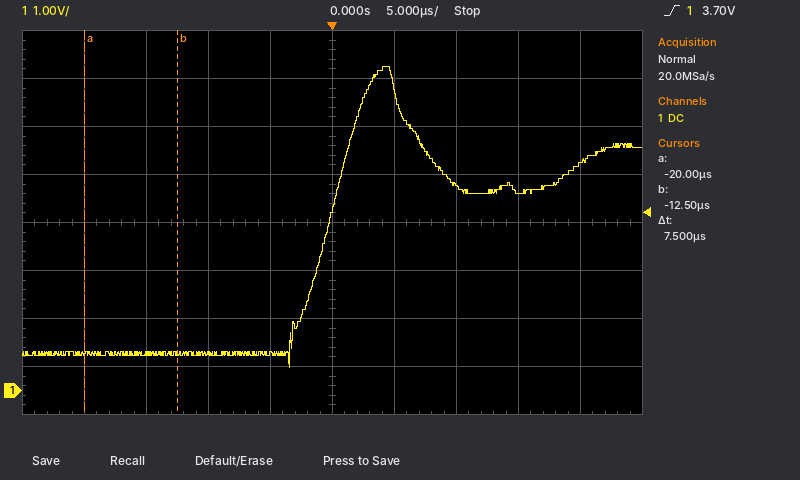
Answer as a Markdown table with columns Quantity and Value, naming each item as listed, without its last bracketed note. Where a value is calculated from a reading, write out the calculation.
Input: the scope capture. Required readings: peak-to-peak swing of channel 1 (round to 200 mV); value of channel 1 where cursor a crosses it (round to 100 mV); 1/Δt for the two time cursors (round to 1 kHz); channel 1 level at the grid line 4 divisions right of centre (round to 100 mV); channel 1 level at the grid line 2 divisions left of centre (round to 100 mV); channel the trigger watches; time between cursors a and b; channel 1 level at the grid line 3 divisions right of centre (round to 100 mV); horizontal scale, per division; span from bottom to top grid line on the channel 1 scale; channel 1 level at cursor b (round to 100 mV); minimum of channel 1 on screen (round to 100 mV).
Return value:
| Quantity | Value |
|---|---|
| peak-to-peak swing of channel 1 | 6.2 V |
| value of channel 1 where cursor a crosses it | 800 mV |
| 1/Δt for the two time cursors | 1 / 7.5 µs ≈ 133 kHz |
| channel 1 level at the grid line 4 divisions right of centre | 4.7 V |
| channel 1 level at the grid line 2 divisions left of centre | 800 mV |
| channel the trigger watches | channel 1 |
| time between cursors a and b | 7.5 µs |
| channel 1 level at the grid line 3 divisions right of centre | 4.1 V |
| horizontal scale, per division | 5 µs |
| span from bottom to top grid line on the channel 1 scale | 8 V |
| channel 1 level at cursor b | 800 mV |
| minimum of channel 1 on screen | 500 mV |
